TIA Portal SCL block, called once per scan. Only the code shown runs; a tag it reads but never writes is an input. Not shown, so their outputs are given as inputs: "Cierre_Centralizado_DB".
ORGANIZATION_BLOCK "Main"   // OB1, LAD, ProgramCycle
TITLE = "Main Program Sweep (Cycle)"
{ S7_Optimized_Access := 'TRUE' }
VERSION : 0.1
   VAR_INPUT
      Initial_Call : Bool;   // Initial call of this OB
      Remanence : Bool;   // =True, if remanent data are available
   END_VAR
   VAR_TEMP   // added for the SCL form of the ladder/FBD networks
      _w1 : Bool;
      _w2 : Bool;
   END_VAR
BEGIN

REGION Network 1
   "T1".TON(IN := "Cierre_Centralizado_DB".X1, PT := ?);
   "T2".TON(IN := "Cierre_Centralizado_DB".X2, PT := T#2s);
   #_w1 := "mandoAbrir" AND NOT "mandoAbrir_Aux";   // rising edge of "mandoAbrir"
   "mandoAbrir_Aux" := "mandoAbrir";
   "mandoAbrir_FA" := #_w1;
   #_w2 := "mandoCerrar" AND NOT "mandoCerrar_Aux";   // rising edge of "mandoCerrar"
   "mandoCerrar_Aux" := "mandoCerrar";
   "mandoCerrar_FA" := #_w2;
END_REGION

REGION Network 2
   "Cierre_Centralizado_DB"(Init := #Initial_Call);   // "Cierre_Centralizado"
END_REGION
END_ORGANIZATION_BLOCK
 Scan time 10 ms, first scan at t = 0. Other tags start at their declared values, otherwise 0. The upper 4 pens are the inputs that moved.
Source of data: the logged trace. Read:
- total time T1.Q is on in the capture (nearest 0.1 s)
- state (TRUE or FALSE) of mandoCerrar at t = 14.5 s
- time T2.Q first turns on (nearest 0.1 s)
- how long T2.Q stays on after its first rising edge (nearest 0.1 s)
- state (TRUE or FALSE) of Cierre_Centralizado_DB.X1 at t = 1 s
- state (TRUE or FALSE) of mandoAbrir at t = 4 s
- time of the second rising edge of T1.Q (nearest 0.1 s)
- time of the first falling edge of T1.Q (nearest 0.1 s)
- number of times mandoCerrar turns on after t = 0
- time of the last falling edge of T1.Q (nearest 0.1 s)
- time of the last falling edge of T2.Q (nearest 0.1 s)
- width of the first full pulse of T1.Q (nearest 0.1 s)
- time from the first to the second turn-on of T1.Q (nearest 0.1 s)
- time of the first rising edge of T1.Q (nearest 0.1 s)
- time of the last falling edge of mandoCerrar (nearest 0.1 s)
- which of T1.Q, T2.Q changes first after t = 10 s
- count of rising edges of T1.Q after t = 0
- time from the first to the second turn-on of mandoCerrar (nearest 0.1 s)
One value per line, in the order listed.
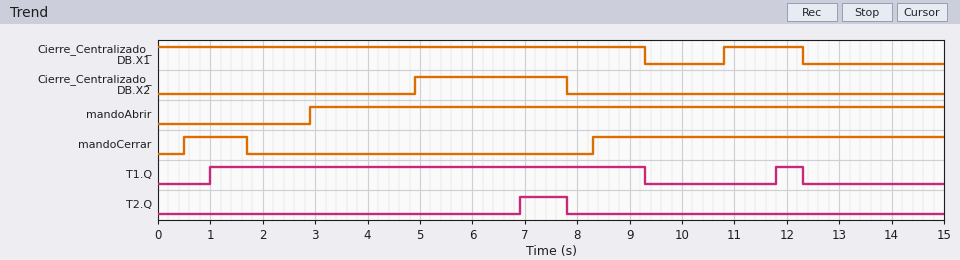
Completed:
8.8 s
TRUE
6.9 s
0.9 s
TRUE
TRUE
11.8 s
9.3 s
2
12.3 s
7.8 s
8.3 s
10.8 s
1.0 s
1.7 s
T1.Q
2
7.8 s
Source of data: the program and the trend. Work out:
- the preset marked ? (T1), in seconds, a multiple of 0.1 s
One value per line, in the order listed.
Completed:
1.0 s
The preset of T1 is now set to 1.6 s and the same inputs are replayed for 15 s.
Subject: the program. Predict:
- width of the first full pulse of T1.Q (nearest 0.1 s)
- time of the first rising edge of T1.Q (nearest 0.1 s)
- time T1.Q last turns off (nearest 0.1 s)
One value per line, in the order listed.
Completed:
7.7 s
1.6 s
9.3 s
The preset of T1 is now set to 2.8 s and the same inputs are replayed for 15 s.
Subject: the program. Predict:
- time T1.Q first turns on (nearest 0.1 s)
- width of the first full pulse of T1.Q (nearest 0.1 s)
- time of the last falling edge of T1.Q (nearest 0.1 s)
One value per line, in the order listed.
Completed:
2.8 s
6.5 s
9.3 s
